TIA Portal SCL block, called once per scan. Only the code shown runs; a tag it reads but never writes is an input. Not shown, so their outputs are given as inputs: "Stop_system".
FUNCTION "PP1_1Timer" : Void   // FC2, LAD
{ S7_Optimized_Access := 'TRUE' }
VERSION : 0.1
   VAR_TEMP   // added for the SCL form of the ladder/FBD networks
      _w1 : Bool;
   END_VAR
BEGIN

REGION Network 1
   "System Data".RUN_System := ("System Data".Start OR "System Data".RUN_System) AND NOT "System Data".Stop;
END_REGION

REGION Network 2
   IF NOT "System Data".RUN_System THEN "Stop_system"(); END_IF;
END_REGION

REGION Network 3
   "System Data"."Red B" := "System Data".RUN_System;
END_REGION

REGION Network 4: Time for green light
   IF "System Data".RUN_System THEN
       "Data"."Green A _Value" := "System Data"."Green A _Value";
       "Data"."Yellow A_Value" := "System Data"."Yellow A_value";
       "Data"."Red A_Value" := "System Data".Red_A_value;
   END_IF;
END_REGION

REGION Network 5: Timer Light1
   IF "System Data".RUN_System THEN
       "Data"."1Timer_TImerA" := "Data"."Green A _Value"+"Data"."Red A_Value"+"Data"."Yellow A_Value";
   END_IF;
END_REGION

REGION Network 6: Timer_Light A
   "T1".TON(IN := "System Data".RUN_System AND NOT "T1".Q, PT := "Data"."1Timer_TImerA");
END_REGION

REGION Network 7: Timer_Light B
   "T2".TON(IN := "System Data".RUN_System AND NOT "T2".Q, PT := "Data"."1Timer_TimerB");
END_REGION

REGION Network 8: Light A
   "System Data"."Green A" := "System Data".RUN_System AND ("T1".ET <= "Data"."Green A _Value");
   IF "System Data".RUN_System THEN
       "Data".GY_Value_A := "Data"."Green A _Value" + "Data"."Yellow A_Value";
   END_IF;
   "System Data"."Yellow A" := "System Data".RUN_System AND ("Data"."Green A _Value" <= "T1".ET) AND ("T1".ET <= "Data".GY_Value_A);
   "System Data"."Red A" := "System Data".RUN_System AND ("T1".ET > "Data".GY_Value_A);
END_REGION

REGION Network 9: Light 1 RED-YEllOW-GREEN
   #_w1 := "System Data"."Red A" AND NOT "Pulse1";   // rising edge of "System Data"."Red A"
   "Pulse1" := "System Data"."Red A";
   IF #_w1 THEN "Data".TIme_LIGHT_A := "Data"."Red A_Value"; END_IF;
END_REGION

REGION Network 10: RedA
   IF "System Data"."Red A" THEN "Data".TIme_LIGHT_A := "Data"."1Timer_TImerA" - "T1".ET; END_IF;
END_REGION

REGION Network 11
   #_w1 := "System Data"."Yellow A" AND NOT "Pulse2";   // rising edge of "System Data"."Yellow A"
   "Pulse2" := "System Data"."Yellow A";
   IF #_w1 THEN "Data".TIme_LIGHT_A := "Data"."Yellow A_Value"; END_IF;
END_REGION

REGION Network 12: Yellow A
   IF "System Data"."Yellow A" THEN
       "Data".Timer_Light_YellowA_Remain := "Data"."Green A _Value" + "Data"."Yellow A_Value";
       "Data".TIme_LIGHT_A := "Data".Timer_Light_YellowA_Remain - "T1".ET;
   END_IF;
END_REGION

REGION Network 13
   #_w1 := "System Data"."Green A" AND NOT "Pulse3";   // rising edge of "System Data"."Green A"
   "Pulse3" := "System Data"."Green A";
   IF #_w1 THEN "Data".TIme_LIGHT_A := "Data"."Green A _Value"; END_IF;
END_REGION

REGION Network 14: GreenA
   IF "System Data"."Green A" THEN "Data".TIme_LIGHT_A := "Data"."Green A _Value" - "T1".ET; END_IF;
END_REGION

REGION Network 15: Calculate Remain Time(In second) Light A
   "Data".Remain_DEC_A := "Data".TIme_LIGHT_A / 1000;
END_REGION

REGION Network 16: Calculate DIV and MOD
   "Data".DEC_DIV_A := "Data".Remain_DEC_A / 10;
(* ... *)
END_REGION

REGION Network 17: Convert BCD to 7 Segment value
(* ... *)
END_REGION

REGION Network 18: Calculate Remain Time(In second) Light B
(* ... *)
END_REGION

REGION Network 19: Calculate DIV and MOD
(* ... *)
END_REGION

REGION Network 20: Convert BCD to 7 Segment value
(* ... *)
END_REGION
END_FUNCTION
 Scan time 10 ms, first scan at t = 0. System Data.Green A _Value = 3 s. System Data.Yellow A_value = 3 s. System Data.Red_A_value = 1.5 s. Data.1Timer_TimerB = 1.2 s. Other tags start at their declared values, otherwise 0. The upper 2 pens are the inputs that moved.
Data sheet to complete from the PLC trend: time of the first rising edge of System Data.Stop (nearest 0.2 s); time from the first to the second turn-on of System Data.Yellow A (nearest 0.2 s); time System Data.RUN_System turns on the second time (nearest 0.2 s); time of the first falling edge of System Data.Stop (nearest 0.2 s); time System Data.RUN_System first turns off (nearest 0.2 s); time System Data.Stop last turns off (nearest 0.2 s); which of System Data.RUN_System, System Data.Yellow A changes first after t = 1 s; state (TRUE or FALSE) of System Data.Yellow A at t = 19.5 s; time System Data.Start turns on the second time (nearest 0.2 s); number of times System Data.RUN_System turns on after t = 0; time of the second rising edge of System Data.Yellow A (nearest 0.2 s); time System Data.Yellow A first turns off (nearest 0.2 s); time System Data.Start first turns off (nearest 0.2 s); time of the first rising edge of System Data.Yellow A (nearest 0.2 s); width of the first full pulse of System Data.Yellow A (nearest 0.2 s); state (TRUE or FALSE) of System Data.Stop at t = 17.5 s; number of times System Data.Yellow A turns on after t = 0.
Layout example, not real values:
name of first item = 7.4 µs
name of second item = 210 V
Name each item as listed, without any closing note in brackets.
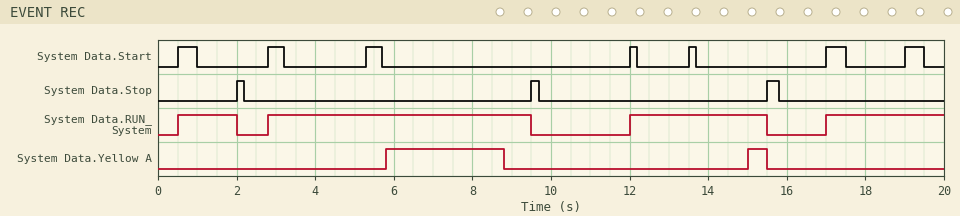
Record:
time of the first rising edge of System Data.Stop = 2.0 s
time from the first to the second turn-on of System Data.Yellow A = 9.2 s
time System Data.RUN_System turns on the second time = 2.8 s
time of the first falling edge of System Data.Stop = 2.2 s
time System Data.RUN_System first turns off = 2.0 s
time System Data.Stop last turns off = 15.8 s
which of System Data.RUN_System, System Data.Yellow A changes first after t = 1 s = System Data.RUN_System
state (TRUE or FALSE) of System Data.Yellow A at t = 19.5 s = FALSE
time System Data.Start turns on the second time = 2.8 s
number of times System Data.RUN_System turns on after t = 0 = 4
time of the second rising edge of System Data.Yellow A = 15.0 s
time System Data.Yellow A first turns off = 8.8 s
time System Data.Start first turns off = 1.0 s
time of the first rising edge of System Data.Yellow A = 5.8 s
width of the first full pulse of System Data.Yellow A = 3.0 s
state (TRUE or FALSE) of System Data.Stop at t = 17.5 s = FALSE
number of times System Data.Yellow A turns on after t = 0 = 2
